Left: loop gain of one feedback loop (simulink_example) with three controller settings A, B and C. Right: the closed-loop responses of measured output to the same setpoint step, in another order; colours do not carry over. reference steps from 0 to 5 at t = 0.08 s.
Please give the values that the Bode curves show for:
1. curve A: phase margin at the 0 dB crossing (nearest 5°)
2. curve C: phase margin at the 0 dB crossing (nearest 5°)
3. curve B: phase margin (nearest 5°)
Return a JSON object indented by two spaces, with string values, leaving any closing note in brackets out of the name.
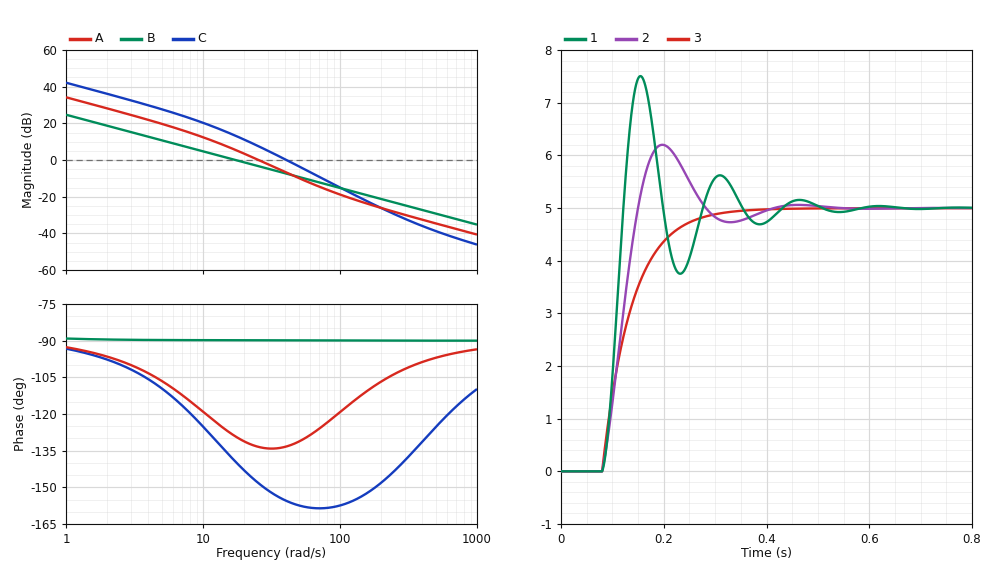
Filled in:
{
  "curve A: phase margin at the 0 dB crossing": "45°",
  "curve C: phase margin at the 0 dB crossing": "25°",
  "curve B: phase margin": "90°"
}
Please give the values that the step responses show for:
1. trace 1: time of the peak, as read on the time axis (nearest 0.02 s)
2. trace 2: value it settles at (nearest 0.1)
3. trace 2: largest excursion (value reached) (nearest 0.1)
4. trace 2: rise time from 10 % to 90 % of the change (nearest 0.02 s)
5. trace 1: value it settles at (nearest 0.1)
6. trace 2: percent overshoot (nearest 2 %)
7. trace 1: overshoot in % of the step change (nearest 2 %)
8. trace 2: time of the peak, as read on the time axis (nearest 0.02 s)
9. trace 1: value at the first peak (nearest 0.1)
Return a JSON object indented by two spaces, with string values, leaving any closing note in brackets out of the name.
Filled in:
{
  "trace 1: time of the peak, as read on the time axis": "0.16 s",
  "trace 2: value it settles at": "5.0",
  "trace 2: largest excursion (value reached)": "6.2",
  "trace 2: rise time from 10 % to 90 % of the change": "0.06 s",
  "trace 1: value it settles at": "5.0",
  "trace 2: percent overshoot": "24 %",
  "trace 1: overshoot in % of the step change": "50 %",
  "trace 2: time of the peak, as read on the time axis": "0.20 s",
  "trace 1: value at the first peak": "7.5"
}
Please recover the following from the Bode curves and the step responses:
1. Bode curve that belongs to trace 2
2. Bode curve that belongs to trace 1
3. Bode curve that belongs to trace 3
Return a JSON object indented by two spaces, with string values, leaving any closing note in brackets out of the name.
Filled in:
{
  "Bode curve that belongs to trace 2": "A",
  "Bode curve that belongs to trace 1": "C",
  "Bode curve that belongs to trace 3": "B"
}
